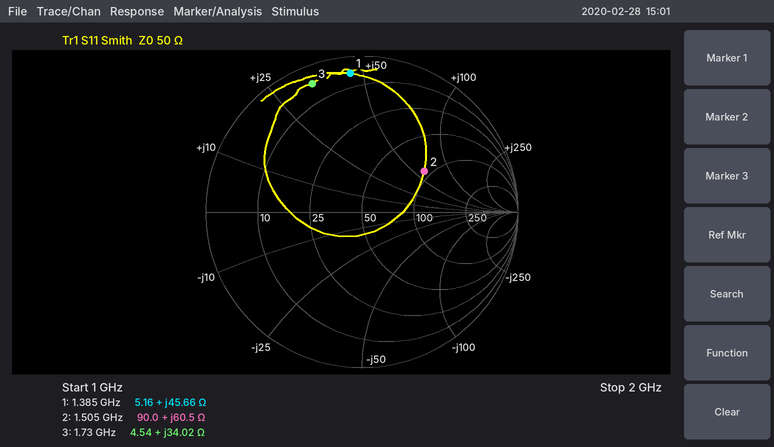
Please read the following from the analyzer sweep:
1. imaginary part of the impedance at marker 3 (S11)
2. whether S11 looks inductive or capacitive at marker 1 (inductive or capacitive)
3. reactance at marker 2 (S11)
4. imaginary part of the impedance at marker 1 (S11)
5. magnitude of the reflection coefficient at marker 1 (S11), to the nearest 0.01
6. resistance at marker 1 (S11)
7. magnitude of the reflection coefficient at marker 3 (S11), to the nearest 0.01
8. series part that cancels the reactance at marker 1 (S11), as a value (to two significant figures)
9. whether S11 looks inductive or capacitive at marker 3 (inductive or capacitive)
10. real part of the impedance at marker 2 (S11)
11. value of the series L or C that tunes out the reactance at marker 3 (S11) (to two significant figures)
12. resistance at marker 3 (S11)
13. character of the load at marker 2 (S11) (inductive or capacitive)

+34.02 Ω
inductive
+60.5 Ω
+45.66 Ω
0.89
5.16 Ω
0.88
2.5 pF
inductive
90.0 Ω
2.7 pF
4.54 Ω
inductive
